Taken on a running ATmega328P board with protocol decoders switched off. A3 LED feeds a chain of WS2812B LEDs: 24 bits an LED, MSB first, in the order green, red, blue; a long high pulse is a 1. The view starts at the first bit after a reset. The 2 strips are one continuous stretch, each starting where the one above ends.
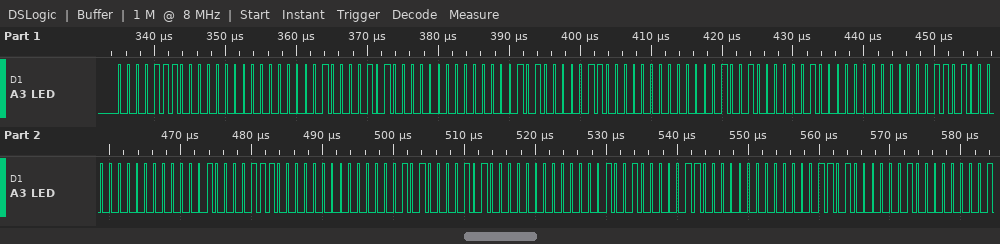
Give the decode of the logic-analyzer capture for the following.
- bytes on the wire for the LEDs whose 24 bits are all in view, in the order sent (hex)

0E 00 01 0A 00 05 06 00 09 02 00 0D 00 01 0E 00 05 0A 00 09 06 00 0D 02
